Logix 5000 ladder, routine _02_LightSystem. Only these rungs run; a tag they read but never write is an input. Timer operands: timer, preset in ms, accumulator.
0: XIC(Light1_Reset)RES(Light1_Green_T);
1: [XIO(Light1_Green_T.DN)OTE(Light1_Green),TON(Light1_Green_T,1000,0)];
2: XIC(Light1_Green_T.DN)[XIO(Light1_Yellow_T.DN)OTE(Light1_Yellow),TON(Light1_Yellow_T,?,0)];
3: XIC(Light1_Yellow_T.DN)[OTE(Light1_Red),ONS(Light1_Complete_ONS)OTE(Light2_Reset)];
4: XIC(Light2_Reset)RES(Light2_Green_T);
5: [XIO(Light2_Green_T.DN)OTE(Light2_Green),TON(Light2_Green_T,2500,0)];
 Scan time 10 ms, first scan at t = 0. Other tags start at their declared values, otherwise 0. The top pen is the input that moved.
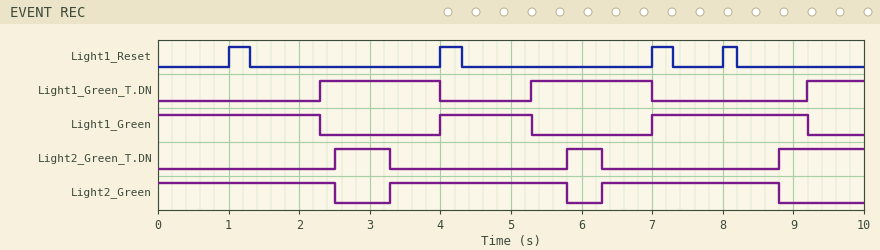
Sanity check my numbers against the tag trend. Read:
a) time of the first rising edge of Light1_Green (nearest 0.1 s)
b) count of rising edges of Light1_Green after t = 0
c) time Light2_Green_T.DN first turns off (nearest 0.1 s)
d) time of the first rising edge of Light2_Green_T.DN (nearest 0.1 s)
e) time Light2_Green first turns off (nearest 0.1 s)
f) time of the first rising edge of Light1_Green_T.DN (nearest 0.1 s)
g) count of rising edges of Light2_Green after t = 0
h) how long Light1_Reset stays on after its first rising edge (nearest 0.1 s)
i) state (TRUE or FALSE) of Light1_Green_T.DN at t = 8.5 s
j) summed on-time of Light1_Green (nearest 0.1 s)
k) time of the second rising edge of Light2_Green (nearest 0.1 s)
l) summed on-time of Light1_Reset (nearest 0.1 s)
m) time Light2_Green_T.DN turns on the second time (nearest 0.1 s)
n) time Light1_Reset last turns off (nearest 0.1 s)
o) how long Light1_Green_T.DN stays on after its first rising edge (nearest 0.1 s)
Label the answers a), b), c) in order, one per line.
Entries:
a) 4.0 s
b) 2
c) 3.3 s
d) 2.5 s
e) 2.5 s
f) 2.3 s
g) 2
h) 0.3 s
i) FALSE
j) 5.8 s
k) 6.3 s
l) 1.1 s
m) 5.8 s
n) 8.2 s
o) 1.7 s
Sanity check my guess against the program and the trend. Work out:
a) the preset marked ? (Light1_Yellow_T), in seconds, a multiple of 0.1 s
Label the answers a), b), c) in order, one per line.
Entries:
a) 1.0 s
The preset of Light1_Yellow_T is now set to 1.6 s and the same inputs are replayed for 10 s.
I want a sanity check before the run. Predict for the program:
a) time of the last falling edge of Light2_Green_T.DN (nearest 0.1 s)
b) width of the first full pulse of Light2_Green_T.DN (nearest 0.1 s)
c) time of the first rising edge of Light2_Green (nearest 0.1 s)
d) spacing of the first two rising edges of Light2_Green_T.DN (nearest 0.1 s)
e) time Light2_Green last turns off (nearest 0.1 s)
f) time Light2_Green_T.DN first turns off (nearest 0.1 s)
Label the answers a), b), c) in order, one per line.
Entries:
a) 6.9 s
b) 1.4 s
c) 3.9 s
d) 3.9 s
e) 9.4 s
f) 3.9 s
